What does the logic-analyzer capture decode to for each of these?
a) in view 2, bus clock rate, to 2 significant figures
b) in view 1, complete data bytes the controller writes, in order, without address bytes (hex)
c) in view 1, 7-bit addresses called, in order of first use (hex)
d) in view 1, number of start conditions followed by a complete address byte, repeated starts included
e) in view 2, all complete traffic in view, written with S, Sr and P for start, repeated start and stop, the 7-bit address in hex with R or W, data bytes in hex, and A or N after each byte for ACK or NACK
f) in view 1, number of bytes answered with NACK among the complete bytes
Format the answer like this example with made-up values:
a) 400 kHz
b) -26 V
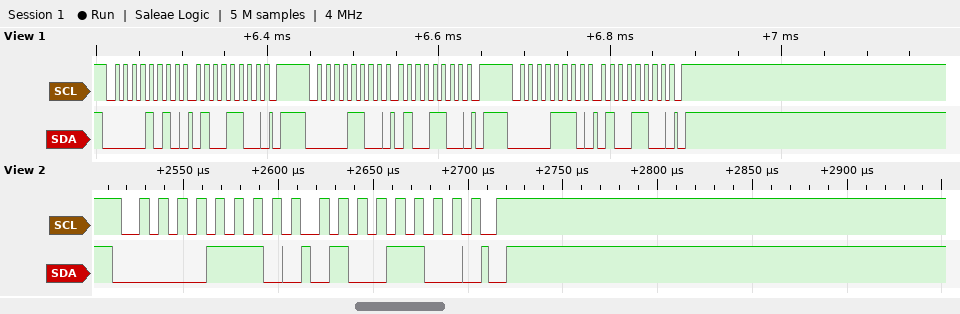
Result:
a) 100 kHz
b) 4C 4C 4C
c) 0x05 0x06 0x07
d) 3
e) S 07W A 4C A P
f) 0
